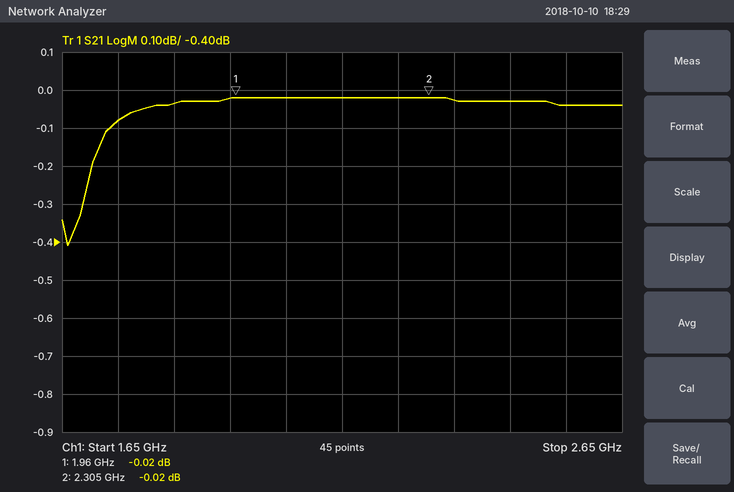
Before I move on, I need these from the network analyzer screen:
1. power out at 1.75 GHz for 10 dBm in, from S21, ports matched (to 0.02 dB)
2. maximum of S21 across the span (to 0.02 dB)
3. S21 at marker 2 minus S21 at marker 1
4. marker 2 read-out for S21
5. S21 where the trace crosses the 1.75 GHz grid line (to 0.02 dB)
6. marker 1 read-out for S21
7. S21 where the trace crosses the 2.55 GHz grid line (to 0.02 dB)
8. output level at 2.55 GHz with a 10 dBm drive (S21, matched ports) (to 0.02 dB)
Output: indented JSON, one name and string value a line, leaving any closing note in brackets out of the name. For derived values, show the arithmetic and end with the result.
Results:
{
  "power out at 1.75 GHz for 10 dBm in, from S21, ports matched": "10 dBm + (-0.08 dB) = 9.92 dBm",
  "maximum of S21 across the span": "-0.02 dB",
  "S21 at marker 2 minus S21 at marker 1": "-0.02 − (-0.02) = 0.00 dB",
  "marker 2 read-out for S21": "-0.02 dB",
  "S21 where the trace crosses the 1.75 GHz grid line": "-0.08 dB",
  "marker 1 read-out for S21": "-0.02 dB",
  "S21 where the trace crosses the 2.55 GHz grid line": "-0.04 dB",
  "output level at 2.55 GHz with a 10 dBm drive (S21, matched ports)": "10 dBm + (-0.04 dB) = 9.96 dBm"
}
